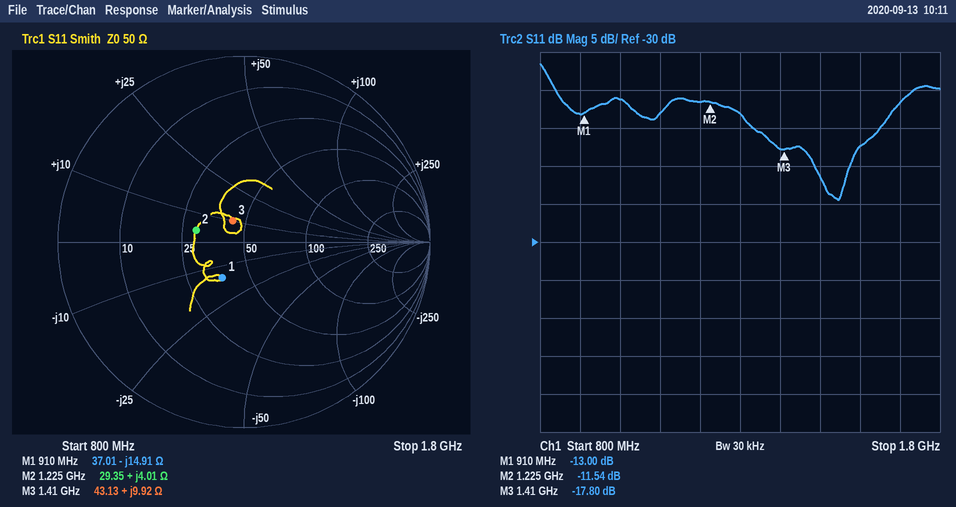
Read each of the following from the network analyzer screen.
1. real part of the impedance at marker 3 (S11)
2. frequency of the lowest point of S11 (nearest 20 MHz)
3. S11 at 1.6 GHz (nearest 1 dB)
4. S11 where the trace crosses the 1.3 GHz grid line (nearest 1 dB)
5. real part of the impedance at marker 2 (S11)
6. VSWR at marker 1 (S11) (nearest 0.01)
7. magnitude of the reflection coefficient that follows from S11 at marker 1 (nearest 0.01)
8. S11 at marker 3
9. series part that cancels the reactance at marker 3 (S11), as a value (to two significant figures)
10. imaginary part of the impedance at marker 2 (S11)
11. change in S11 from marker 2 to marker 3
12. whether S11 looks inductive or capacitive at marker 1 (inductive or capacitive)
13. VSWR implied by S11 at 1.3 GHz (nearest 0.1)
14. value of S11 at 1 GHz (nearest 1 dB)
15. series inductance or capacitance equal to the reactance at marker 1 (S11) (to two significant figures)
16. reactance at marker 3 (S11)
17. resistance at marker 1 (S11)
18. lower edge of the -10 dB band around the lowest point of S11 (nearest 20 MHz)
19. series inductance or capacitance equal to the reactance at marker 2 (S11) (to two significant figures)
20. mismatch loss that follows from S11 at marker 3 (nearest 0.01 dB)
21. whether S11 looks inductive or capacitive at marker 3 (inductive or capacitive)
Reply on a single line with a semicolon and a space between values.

43.13 Ω; 1.54 GHz; -17 dB; -13 dB; 29.35 Ω; 1.58; 0.22; -17.80 dB; 11 pF; +4.01 Ω; -6.26 dB; capacitive; 1.6; -11 dB; 12 pF; +9.92 Ω; 37.01 Ω; 840 MHz; 520 pH; 0.07 dB; inductive
